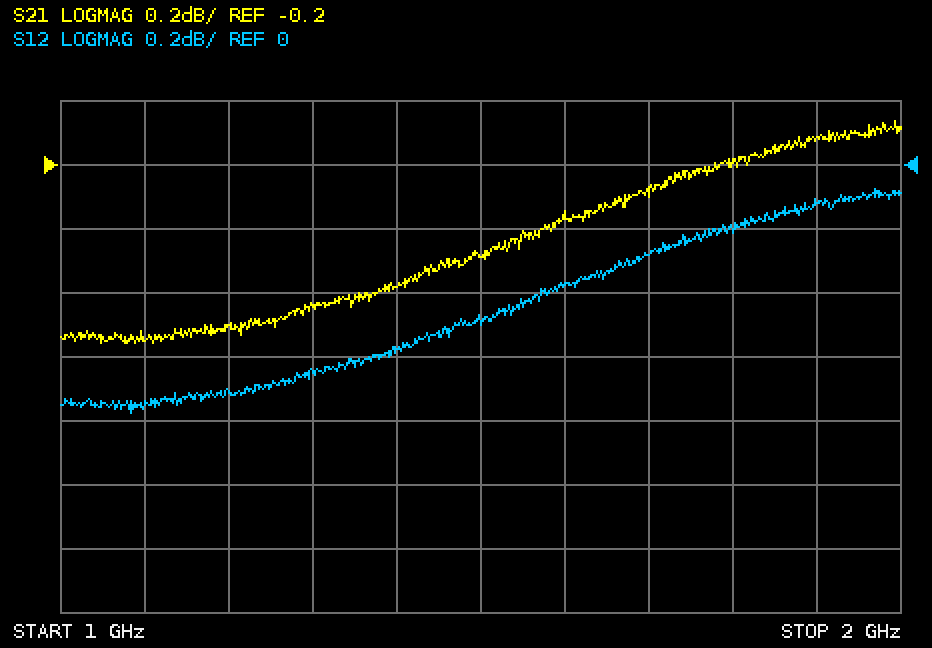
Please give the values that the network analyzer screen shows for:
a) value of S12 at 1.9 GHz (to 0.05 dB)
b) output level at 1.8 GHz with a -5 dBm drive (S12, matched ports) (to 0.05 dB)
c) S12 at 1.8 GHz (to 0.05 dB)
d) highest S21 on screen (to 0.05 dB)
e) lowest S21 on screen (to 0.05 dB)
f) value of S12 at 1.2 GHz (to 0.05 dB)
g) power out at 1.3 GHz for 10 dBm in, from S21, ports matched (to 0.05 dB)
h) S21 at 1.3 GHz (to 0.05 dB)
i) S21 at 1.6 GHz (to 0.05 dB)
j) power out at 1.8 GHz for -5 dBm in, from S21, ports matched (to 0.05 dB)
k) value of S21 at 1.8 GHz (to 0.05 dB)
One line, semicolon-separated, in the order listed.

-0.10 dB; -5.20 dBm; -0.20 dB; -0.05 dB; -0.75 dB; -0.70 dB; 9.35 dBm; -0.65 dB; -0.35 dB; -5.20 dBm; -0.20 dB
